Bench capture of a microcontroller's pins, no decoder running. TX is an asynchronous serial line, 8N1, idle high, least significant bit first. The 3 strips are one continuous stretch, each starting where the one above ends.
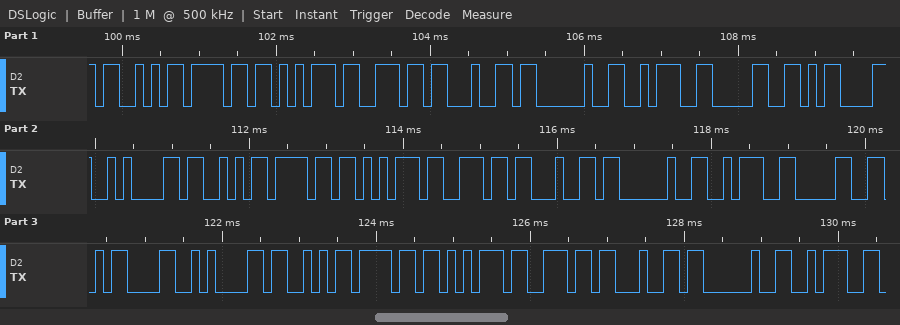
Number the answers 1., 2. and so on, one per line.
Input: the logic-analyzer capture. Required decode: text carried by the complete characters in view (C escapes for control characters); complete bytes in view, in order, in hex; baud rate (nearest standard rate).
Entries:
1. "Sound :0\r\nSound :0\r\nSound :"
2. 53 6F 75 6E 64 20 3A 30 0D 0A 53 6F 75 6E 64 20 3A 30 0D 0A 53 6F 75 6E 64 20 3A
3. 9600 baud
